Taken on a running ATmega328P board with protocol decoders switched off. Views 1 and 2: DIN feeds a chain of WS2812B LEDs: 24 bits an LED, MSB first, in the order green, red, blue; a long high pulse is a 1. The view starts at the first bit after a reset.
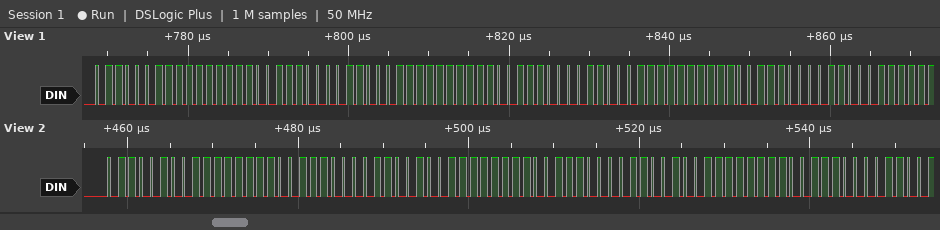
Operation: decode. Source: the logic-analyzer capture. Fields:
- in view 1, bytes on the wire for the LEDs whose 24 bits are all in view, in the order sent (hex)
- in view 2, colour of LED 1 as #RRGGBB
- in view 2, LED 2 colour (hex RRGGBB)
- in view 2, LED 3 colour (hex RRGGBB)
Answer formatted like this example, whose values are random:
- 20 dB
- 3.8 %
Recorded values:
- 63 FF 38 63 FF 38 63 FF 38
- #FF6438
- #FF6438
- #FF6438
